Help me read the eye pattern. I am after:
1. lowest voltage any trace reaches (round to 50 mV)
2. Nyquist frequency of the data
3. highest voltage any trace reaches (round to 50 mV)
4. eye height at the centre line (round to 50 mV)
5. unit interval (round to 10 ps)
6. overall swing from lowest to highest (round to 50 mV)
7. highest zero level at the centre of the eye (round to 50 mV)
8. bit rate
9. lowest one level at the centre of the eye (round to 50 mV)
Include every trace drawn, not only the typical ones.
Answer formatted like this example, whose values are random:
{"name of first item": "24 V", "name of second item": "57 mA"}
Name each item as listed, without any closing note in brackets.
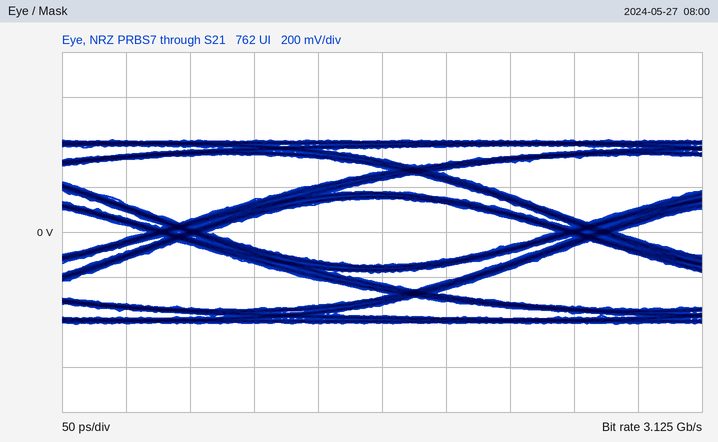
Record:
{"lowest voltage any trace reaches": "-400 mV", "Nyquist frequency of the data": "1.5625 GHz", "highest voltage any trace reaches": "400 mV", "eye height at the centre line": "300 mV", "unit interval": "320 ps", "overall swing from lowest to highest": "800 mV", "highest zero level at the centre of the eye": "-150 mV", "bit rate": "3.125 Gb/s", "lowest one level at the centre of the eye": "150 mV"}
